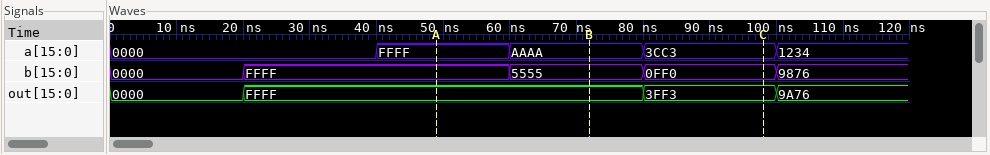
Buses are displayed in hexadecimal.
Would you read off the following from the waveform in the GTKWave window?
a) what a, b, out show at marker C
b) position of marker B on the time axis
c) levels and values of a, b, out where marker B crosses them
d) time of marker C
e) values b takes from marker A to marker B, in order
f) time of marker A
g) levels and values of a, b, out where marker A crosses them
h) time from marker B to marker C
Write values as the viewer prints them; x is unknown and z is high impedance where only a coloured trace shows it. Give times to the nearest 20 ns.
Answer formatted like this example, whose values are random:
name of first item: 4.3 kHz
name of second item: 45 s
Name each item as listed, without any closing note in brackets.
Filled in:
what a, b, out show at marker C: a=3CC3, b=0FF0, out=3FF3
position of marker B on the time axis: 80 ns
levels and values of a, b, out where marker B crosses them: a=AAAA, b=5555, out=FFFF
time of marker C: 100 ns
values b takes from marker A to marker B, in order: FFFF, 5555
time of marker A: 40 ns
levels and values of a, b, out where marker A crosses them: a=FFFF, b=FFFF, out=FFFF
time from marker B to marker C: 20 ns
